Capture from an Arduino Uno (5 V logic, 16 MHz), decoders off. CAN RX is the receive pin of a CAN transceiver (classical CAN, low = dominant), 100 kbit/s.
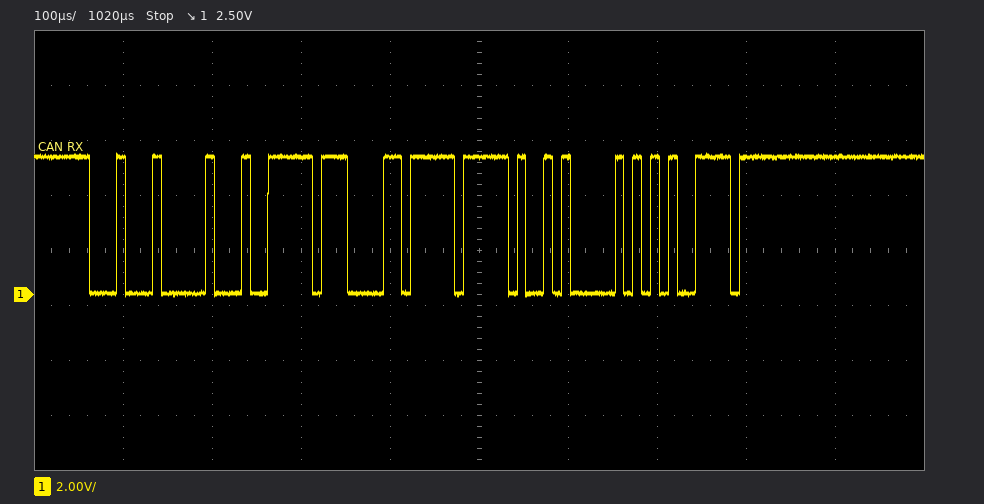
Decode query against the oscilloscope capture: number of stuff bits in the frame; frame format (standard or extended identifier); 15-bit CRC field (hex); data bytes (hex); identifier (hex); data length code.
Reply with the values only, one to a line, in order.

5
standard
0x02A7
FF 0D FF CA
0x110
4
